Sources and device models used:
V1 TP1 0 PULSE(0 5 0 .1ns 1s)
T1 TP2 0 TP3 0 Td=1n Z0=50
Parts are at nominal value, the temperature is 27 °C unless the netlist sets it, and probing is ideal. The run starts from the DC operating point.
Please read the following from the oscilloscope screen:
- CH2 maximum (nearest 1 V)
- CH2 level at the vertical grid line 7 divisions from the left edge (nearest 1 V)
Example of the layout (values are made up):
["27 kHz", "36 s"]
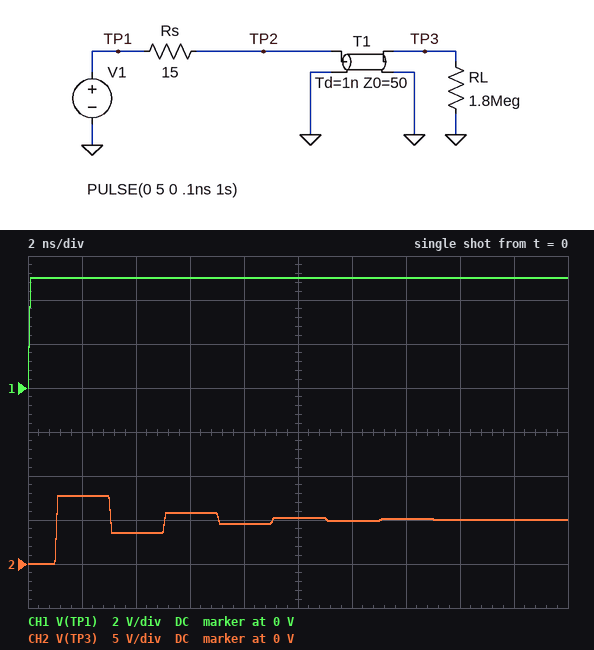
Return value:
["8 V", "5 V"]
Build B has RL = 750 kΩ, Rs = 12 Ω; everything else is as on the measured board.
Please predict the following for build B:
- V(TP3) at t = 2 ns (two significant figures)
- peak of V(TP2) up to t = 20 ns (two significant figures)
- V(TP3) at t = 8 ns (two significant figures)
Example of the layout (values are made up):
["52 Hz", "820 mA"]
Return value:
["8.1 V", "5.6 V", "4.3 V"]
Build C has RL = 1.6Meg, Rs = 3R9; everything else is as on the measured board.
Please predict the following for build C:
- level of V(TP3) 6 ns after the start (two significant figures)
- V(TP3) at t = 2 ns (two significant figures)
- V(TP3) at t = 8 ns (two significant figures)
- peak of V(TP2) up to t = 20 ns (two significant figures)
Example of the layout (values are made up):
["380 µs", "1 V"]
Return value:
["8.1 V", "9.3 V", "2.3 V", "5.3 V"]
